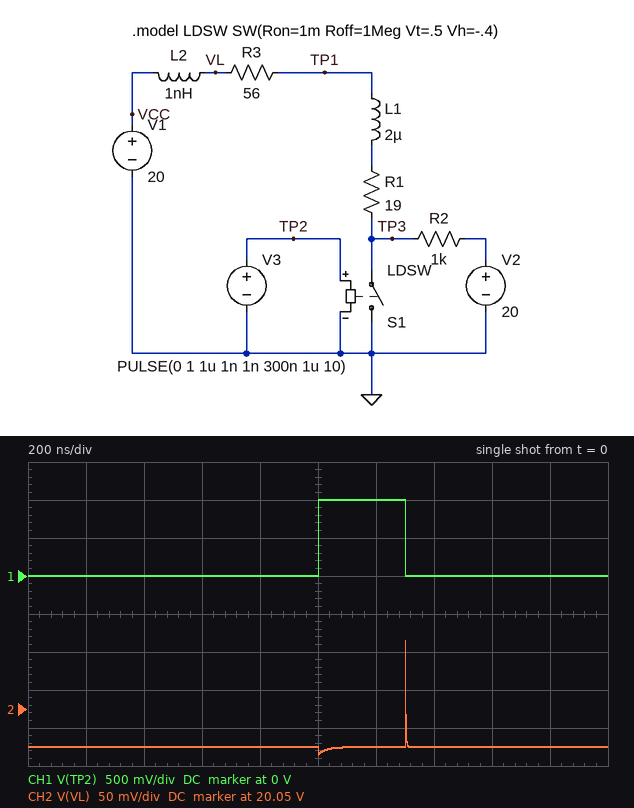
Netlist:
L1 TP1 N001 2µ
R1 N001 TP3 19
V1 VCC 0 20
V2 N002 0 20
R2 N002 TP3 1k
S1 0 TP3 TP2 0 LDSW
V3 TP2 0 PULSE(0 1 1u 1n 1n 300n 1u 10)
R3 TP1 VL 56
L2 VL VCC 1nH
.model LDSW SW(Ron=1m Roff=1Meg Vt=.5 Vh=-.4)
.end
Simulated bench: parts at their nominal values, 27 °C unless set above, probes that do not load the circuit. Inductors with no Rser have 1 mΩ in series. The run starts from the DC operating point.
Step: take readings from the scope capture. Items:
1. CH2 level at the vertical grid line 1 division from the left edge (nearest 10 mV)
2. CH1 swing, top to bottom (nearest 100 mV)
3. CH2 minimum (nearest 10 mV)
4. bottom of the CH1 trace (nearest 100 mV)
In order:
20.00 V
1.0 V
19.99 V
0 V
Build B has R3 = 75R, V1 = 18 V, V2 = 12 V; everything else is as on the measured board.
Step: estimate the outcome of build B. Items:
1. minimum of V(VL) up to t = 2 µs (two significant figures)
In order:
18 V
